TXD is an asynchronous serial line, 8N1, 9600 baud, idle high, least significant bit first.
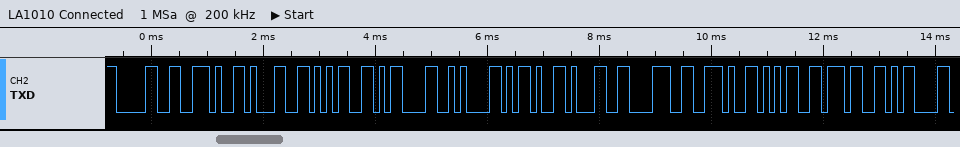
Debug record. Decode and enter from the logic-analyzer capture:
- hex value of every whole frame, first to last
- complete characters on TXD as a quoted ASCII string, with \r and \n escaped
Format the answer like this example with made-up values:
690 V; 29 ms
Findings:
0x30 0x2E 0x31 0x35 0x0D 0x0A 0x2D 0x31 0x38 0x2E 0x35 0x37 0x0D; "0.15\r\n-18.57\r"
